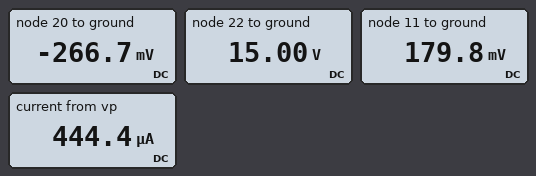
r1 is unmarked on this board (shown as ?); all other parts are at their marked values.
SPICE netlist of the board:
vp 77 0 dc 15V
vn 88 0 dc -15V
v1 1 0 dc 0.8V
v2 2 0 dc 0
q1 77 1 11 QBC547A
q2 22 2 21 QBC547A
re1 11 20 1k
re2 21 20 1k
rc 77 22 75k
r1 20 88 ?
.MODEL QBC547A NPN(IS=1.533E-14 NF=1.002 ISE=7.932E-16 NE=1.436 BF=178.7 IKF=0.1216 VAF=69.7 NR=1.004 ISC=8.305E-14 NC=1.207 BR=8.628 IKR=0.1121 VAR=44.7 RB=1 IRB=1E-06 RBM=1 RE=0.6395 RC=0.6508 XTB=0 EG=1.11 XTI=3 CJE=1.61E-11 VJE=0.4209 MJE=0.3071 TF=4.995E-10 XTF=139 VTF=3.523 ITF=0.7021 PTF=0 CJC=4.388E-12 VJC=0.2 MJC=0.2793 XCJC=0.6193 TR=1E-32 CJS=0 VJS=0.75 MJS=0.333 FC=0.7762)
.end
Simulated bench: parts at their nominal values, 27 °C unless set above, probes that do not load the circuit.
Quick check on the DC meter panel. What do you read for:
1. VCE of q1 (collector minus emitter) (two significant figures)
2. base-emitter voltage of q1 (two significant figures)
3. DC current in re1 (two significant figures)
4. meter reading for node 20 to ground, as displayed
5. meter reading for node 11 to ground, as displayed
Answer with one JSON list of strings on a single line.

["15 V", "620 mV", "450 µA", "-266.7 mV", "179.8 mV"]
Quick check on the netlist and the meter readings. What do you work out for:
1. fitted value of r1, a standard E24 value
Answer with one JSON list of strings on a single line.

["33 kΩ"]
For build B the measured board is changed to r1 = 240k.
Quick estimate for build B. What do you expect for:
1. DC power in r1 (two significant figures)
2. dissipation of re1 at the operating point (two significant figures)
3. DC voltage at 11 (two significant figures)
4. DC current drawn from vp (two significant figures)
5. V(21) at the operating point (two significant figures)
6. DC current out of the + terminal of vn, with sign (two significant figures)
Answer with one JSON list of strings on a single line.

["960 µW", "4.0 µW", "230 mV", "63 µA", "170 mV", "-63 µA"]
